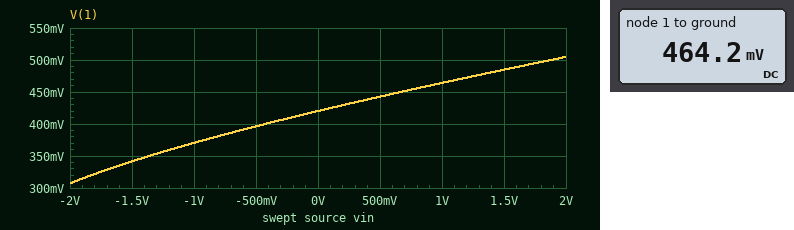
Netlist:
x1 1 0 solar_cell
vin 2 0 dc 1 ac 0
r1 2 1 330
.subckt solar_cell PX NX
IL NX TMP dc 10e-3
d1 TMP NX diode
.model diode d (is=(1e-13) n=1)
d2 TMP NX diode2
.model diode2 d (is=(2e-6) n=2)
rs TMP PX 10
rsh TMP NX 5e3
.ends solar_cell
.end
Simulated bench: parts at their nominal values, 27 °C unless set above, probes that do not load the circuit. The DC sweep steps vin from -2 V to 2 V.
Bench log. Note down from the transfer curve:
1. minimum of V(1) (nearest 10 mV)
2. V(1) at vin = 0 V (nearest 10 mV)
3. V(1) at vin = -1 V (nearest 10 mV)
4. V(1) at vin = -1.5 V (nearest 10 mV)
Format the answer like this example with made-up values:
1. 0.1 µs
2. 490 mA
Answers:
1. 310 mV
2. 420 mV
3. 370 mV
4. 340 mV
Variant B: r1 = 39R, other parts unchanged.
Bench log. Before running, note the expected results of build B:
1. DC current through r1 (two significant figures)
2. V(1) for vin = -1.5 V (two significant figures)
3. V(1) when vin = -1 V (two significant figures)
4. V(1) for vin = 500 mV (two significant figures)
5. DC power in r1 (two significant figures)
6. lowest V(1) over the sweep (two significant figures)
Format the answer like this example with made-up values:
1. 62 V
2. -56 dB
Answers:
1. 11 mA
2. -1.1 V
3. -610 mV
4. 460 mV
5. 4.4 mW
6. -1.6 V
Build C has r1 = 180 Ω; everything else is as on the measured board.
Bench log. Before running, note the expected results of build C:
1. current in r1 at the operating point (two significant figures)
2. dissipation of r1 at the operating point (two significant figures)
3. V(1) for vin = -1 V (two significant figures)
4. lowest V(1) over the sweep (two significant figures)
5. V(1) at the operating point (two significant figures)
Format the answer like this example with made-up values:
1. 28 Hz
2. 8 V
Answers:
1. 2.9 mA
2. 1.5 mW
3. 300 mV
4. -200 mV
5. 480 mV
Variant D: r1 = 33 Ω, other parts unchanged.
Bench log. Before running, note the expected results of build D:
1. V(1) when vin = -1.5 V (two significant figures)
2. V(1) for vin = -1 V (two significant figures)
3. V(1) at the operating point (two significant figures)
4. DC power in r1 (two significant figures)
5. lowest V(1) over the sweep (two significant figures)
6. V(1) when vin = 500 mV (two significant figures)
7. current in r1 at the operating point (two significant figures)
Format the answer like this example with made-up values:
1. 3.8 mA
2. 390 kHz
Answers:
1. -1.2 V
2. -670 mV
3. 600 mV
4. 4.8 mW
5. -1.7 V
6. 460 mV
7. 12 mA
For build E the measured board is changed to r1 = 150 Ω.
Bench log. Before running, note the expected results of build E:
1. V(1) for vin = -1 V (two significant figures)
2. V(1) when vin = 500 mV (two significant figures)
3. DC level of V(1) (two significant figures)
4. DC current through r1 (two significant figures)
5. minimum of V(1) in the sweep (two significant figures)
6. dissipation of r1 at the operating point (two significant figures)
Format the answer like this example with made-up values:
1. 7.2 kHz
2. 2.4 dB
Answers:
1. 260 mV
2. 450 mV
3. 490 mV
4. 3.4 mA
5. -490 mV
6. 1.7 mW
